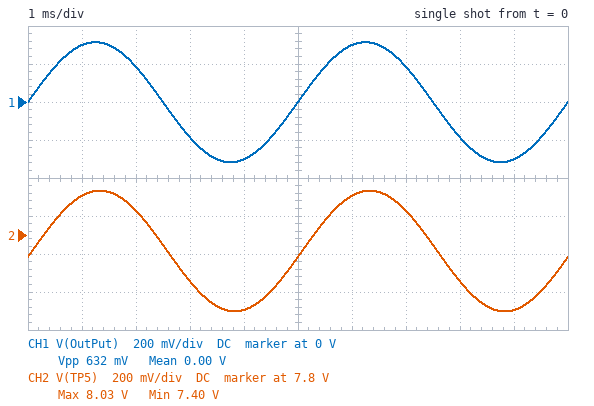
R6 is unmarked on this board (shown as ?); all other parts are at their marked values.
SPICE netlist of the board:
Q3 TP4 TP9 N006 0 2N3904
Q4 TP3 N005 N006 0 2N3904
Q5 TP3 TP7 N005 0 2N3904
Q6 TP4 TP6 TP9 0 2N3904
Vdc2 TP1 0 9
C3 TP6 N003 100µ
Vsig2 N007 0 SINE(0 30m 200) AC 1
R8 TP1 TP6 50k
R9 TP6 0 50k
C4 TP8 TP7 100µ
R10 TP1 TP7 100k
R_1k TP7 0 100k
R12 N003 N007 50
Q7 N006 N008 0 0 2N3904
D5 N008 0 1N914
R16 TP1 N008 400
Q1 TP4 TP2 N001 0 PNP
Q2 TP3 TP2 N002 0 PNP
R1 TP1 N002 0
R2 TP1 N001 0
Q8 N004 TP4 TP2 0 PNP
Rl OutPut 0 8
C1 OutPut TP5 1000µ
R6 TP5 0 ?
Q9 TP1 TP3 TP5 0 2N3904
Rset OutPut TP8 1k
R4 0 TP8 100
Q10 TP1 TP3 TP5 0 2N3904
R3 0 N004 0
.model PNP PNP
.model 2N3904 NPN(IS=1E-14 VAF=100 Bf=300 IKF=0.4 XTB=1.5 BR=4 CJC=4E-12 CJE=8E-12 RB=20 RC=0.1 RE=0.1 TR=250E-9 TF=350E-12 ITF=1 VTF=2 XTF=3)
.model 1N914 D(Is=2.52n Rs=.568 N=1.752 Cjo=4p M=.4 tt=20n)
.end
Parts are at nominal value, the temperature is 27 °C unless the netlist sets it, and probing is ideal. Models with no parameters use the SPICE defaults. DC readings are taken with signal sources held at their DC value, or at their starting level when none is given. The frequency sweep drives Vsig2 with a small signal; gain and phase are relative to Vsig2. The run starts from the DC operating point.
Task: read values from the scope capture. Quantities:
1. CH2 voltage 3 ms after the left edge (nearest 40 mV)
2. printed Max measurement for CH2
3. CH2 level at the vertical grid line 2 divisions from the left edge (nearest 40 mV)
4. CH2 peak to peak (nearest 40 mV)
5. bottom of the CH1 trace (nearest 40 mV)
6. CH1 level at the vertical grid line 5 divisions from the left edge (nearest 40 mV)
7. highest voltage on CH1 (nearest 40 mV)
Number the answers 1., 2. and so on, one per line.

1. 7.56 V
2. 8.03 V
3. 7.92 V
4. 640 mV
5. -320 mV
6. 0 V
7. 320 mV
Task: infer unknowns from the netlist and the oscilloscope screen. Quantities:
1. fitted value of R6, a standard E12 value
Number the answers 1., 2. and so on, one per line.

1. 120 Ω
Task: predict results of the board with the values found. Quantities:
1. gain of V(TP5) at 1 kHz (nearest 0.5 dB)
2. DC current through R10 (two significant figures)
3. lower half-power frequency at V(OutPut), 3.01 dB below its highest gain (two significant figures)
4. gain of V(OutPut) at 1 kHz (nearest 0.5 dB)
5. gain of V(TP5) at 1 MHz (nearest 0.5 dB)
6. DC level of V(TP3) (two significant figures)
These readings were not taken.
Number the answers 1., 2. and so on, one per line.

1. 20.5 dB
2. 45 µA
3. 190 mHz
4. 20.5 dB
5. 20.5 dB
6. 8.4 V
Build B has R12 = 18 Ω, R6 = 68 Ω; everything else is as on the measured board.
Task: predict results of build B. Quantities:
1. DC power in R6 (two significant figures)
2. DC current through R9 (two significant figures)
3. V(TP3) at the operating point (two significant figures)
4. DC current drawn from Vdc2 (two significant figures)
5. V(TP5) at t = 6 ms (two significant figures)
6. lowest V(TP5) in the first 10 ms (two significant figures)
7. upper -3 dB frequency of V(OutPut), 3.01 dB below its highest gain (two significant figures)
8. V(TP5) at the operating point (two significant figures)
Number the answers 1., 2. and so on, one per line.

1. 650 mW
2. 90 µA
3. 7.4 V
4. 140 mA
5. 7.0 V
6. 6.4 V
7. 5.0 MHz
8. 6.7 V
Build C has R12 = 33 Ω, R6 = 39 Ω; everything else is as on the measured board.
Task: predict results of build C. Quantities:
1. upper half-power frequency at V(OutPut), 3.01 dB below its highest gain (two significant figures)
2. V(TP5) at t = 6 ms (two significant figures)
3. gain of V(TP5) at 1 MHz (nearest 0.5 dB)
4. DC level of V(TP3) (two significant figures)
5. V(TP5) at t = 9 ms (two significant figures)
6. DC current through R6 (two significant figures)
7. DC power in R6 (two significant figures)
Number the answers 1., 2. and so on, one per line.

1. 4.6 MHz
2. 5.7 V
3. 20.0 dB
4. 6.2 V
5. 5.1 V
6. 140 mA
7. 750 mW
